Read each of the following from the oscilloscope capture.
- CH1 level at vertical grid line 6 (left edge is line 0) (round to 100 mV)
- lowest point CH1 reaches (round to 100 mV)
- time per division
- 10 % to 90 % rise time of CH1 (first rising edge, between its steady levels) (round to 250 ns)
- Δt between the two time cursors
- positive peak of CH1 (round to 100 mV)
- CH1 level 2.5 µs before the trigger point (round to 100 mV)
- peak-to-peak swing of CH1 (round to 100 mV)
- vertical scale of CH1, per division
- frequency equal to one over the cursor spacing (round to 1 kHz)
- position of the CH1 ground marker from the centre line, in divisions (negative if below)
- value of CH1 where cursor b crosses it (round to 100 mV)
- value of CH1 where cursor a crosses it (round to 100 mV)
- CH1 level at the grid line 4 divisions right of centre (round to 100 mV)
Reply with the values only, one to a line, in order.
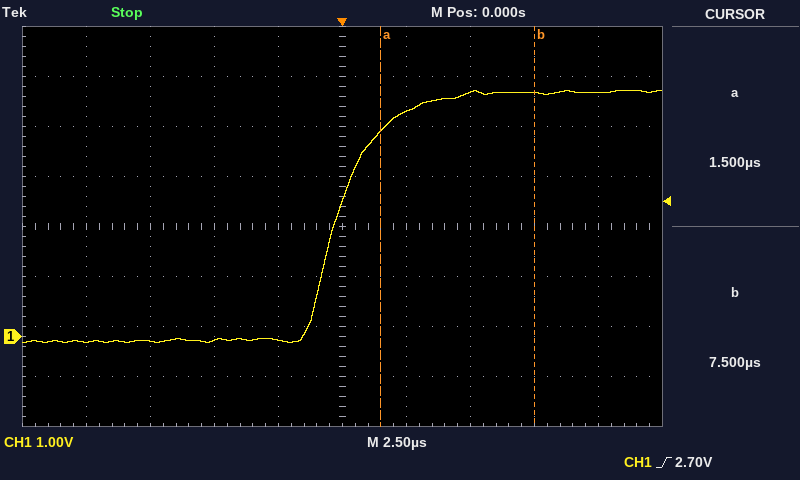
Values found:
4.5 V
-100 mV
2.5 µs
3.25 µs
6.00 µs
4.9 V
-100 mV
5.0 V
1 V
167 kHz
-2.2 div
4.9 V
4.1 V
4.9 V
